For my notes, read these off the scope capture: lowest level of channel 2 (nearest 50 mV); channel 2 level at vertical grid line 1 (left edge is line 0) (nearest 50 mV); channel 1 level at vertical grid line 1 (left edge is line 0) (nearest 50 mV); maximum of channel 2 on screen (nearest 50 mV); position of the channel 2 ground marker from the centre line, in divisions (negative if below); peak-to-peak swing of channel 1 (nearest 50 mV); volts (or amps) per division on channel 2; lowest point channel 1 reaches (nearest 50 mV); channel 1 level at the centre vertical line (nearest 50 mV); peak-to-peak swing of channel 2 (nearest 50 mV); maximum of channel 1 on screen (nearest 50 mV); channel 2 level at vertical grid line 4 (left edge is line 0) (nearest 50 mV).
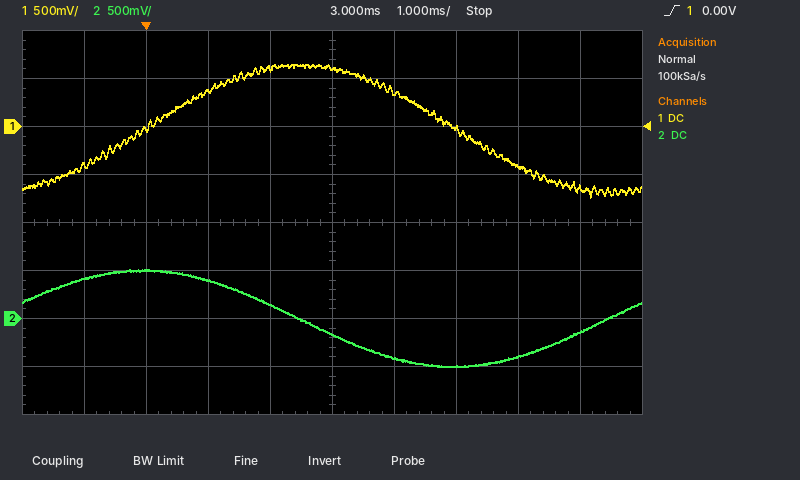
-500 mV
400 mV
-400 mV
500 mV
-2.0 div
1.40 V
500 mV
-750 mV
600 mV
1.00 V
650 mV
150 mV
